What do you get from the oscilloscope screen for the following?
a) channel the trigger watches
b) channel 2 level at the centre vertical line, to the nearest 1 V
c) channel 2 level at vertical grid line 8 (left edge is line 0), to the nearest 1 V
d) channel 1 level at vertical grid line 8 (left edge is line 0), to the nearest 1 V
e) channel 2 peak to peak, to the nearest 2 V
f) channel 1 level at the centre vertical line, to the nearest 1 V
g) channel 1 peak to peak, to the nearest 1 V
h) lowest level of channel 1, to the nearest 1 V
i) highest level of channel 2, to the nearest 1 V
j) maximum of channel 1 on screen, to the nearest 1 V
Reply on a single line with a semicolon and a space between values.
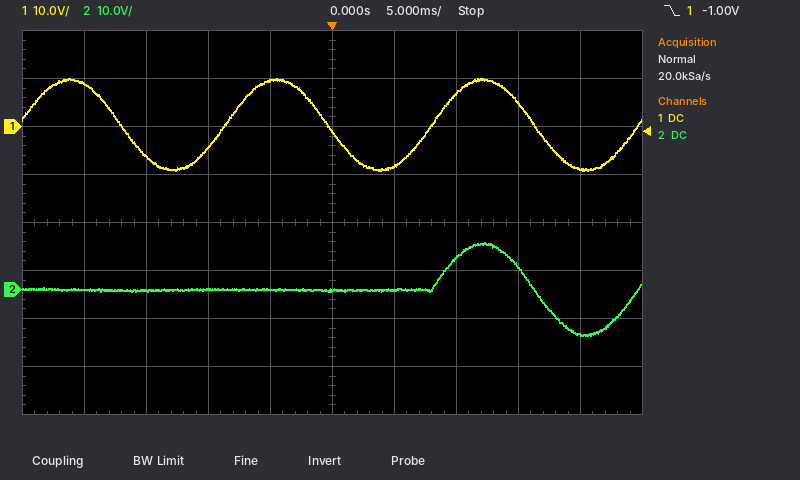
channel 1; 0 V; 5 V; 5 V; 20 V; -1 V; 19 V; -9 V; 10 V; 10 V
